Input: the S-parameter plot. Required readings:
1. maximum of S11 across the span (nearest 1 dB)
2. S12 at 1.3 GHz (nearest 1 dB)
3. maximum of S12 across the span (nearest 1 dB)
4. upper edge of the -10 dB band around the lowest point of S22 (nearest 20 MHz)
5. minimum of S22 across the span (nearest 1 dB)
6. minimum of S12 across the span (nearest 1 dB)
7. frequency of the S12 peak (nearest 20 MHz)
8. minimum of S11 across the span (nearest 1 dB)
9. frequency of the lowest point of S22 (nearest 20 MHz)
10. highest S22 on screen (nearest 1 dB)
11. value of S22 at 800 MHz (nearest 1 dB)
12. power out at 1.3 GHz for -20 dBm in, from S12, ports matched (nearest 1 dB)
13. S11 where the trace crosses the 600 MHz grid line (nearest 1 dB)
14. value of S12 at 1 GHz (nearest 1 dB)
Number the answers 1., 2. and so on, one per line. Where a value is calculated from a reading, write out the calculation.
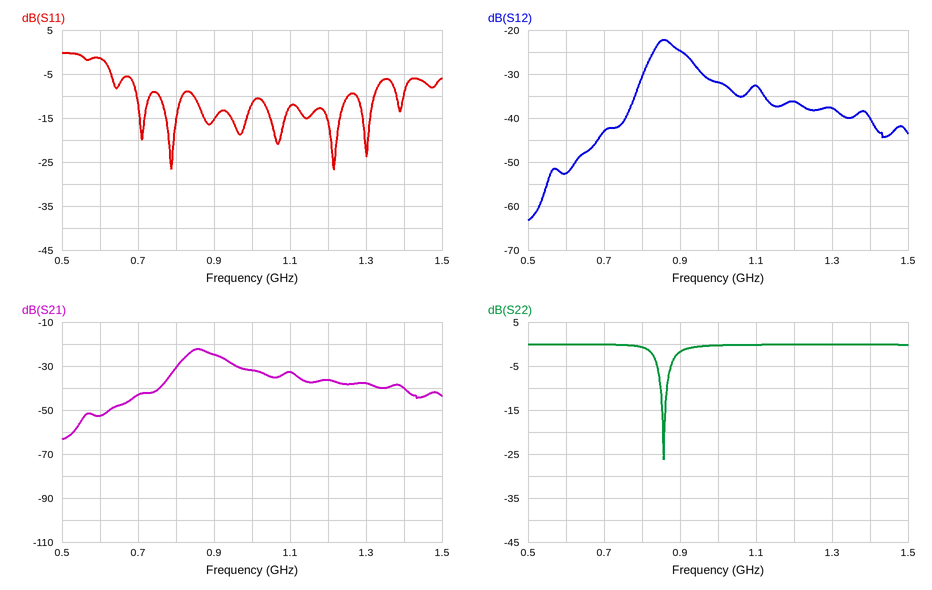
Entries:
1. 0 dB
2. -38 dB
3. -22 dB
4. 860 MHz
5. -26 dB
6. -63 dB
7. 860 MHz
8. -27 dB
9. 860 MHz
10. 0 dB
11. -1 dB
12. -20 dBm + (-38 dB) = -58 dBm
13. -1 dB
14. -32 dB
